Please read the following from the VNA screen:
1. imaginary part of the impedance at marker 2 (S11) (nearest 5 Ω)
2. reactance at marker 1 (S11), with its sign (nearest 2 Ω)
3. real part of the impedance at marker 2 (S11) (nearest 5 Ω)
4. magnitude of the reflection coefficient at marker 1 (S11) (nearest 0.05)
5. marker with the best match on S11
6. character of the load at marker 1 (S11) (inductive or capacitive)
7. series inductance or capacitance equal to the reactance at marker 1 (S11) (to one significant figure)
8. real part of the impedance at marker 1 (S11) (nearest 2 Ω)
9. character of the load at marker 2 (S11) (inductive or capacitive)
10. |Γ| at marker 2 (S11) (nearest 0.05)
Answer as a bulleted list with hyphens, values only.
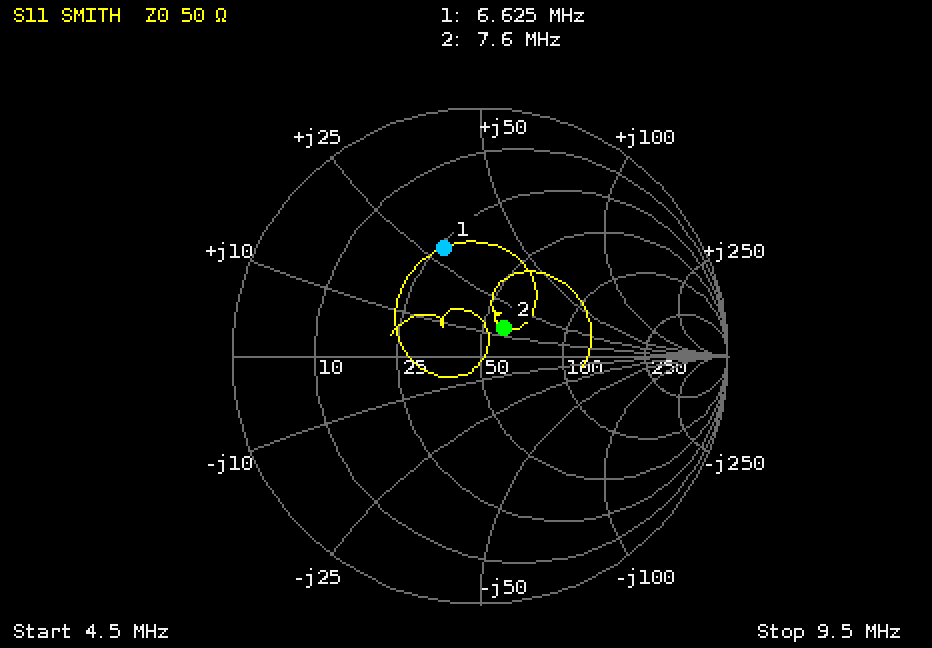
- +15 Ω
- +30 Ω
- 60 Ω
- 0.45
- marker 2
- inductive
- 700 nH
- 26 Ω
- inductive
- 0.15
